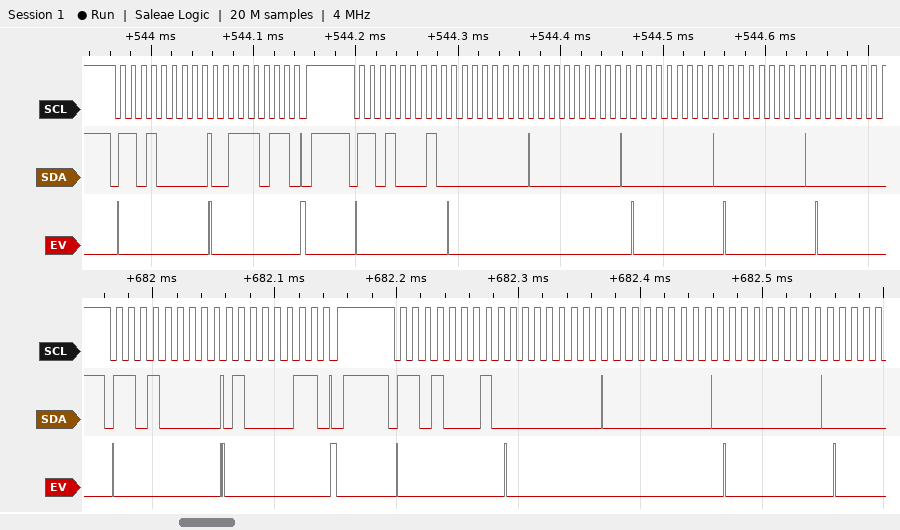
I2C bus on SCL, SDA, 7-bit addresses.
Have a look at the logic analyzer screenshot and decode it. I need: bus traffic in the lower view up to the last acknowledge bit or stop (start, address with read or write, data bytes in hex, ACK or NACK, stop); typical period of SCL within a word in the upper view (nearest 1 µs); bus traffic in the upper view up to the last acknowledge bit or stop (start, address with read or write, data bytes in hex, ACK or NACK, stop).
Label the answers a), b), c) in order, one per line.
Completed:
a) start, address 68 write ACK, 43 ACK, stop, start, address 68 read ACK, 00 ACK, 00 ACK, 00 ACK
b) 10 µs
c) start, address 68 write ACK, 3B ACK, stop, start, address 68 read ACK, 00 ACK, 00 ACK, 00 ACK, 00 ACK
